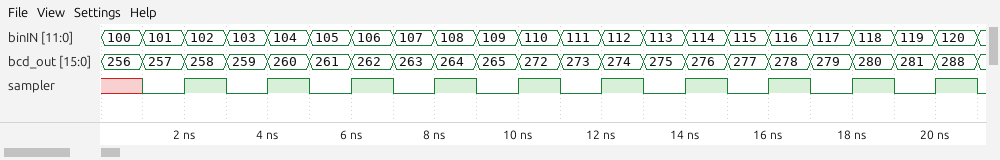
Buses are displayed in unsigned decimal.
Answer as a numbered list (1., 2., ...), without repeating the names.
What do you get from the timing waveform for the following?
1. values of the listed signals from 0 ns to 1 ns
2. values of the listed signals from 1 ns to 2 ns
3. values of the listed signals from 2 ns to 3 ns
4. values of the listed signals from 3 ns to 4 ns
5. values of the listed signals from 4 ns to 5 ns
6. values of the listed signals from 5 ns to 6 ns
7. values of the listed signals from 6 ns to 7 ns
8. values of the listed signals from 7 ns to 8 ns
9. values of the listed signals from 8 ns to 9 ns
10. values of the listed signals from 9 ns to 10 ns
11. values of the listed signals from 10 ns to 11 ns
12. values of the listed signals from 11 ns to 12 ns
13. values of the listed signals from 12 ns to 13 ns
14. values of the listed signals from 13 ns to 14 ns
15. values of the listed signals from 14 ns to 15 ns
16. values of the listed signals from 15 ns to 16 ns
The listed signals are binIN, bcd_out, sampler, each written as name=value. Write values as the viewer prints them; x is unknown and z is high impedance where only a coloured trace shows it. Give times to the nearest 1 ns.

1. binIN=100, bcd_out=256, sampler=x
2. binIN=101, bcd_out=257, sampler=0
3. binIN=102, bcd_out=258, sampler=1
4. binIN=103, bcd_out=259, sampler=0
5. binIN=104, bcd_out=260, sampler=1
6. binIN=105, bcd_out=261, sampler=0
7. binIN=106, bcd_out=262, sampler=1
8. binIN=107, bcd_out=263, sampler=0
9. binIN=108, bcd_out=264, sampler=1
10. binIN=109, bcd_out=265, sampler=0
11. binIN=110, bcd_out=272, sampler=1
12. binIN=111, bcd_out=273, sampler=0
13. binIN=112, bcd_out=274, sampler=1
14. binIN=113, bcd_out=275, sampler=0
15. binIN=114, bcd_out=276, sampler=1
16. binIN=115, bcd_out=277, sampler=0
